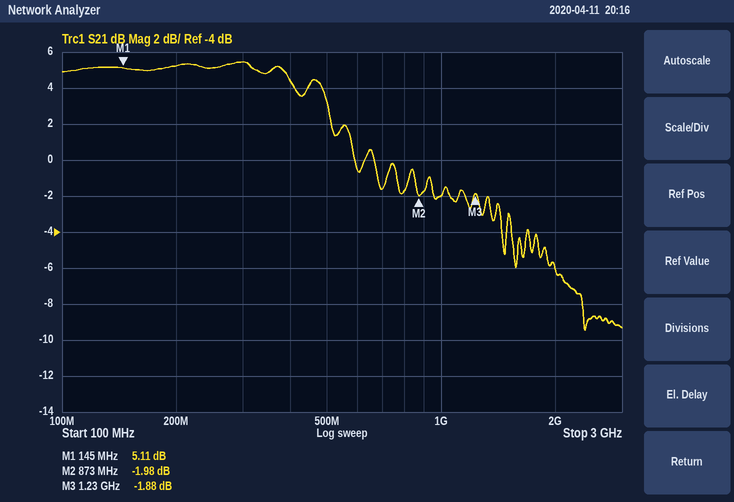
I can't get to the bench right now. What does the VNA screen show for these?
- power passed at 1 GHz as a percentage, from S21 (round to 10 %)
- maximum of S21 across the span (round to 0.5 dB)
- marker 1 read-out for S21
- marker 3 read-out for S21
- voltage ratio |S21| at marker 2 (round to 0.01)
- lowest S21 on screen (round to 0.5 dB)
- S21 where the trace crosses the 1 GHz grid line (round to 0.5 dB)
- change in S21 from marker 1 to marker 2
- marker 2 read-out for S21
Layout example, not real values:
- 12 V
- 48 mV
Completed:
- 60 %
- 5.5 dB
- 5.11 dB
- -1.88 dB
- 0.80
- -9.5 dB
- -2.0 dB
- -7.09 dB
- -1.98 dB
